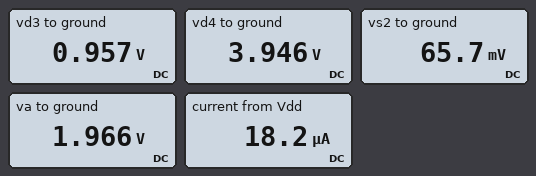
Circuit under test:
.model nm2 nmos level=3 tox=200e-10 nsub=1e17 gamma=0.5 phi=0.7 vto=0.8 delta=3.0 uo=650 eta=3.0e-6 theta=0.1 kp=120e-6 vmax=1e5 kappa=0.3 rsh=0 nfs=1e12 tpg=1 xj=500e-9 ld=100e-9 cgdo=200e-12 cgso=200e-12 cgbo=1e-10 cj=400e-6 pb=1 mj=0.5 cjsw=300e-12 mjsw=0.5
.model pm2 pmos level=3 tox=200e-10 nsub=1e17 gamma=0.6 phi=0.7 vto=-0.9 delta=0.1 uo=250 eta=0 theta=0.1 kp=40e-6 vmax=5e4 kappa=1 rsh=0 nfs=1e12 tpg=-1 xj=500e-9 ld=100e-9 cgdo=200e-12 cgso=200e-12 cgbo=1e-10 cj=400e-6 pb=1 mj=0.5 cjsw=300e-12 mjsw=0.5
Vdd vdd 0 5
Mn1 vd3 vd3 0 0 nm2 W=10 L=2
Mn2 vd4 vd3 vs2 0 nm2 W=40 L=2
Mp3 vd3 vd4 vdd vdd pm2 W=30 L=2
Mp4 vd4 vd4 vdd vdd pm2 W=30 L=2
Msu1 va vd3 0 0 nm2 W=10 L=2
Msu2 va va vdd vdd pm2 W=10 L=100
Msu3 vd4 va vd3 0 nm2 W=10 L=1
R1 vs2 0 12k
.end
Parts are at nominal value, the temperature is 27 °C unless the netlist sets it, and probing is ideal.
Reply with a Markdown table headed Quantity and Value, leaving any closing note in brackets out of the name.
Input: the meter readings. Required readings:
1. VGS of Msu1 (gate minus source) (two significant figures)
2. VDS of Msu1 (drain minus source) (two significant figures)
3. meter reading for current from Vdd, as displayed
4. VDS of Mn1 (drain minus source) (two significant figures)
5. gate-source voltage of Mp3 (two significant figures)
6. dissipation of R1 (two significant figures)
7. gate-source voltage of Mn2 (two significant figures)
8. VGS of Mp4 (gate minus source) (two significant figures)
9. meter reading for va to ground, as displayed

| Quantity | Value |
|---|---|
| VGS of Msu1 (gate minus source) | 960 mV |
| VDS of Msu1 (drain minus source) | 2.0 V |
| meter reading for current from Vdd, as displayed | 18.2 µA |
| VDS of Mn1 (drain minus source) | 960 mV |
| gate-source voltage of Mp3 | -1.1 V |
| dissipation of R1 | 360 nW |
| gate-source voltage of Mn2 | 890 mV |
| VGS of Mp4 (gate minus source) | -1.1 V |
| meter reading for va to ground, as displayed | 1.966 V |
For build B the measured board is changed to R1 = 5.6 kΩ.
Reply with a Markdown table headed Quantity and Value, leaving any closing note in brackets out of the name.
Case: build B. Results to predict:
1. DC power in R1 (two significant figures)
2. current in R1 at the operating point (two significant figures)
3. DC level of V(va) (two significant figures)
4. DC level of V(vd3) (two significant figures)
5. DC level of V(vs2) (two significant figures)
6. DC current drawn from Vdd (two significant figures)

| Quantity | Value |
|---|---|
| DC power in R1 | 2.1 µW |
| current in R1 at the operating point | 19 µA |
| DC level of V(va) | 190 mV |
| DC level of V(vd3) | 1.1 V |
| DC level of V(vs2) | 110 mV |
| DC current drawn from Vdd | 57 µA |
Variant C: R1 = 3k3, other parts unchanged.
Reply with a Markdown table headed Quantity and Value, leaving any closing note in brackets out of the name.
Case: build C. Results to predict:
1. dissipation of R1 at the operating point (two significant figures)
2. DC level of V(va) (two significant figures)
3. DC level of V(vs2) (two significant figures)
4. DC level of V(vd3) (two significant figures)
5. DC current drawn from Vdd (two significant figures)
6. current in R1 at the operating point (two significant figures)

| Quantity | Value |
|---|---|
| dissipation of R1 at the operating point | 11 µW |
| DC level of V(va) | 78 mV |
| DC level of V(vs2) | 190 mV |
| DC level of V(vd3) | 1.3 V |
| DC current drawn from Vdd | 140 µA |
| current in R1 at the operating point | 58 µA |
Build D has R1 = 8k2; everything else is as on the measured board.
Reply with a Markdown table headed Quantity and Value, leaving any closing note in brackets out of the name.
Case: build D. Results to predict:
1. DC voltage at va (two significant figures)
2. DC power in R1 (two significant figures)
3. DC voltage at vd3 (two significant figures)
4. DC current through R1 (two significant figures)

| Quantity | Value |
|---|---|
| DC voltage at va | 1.5 V |
| DC power in R1 | 640 nW |
| DC voltage at vd3 | 990 mV |
| DC current through R1 | 8.8 µA |
